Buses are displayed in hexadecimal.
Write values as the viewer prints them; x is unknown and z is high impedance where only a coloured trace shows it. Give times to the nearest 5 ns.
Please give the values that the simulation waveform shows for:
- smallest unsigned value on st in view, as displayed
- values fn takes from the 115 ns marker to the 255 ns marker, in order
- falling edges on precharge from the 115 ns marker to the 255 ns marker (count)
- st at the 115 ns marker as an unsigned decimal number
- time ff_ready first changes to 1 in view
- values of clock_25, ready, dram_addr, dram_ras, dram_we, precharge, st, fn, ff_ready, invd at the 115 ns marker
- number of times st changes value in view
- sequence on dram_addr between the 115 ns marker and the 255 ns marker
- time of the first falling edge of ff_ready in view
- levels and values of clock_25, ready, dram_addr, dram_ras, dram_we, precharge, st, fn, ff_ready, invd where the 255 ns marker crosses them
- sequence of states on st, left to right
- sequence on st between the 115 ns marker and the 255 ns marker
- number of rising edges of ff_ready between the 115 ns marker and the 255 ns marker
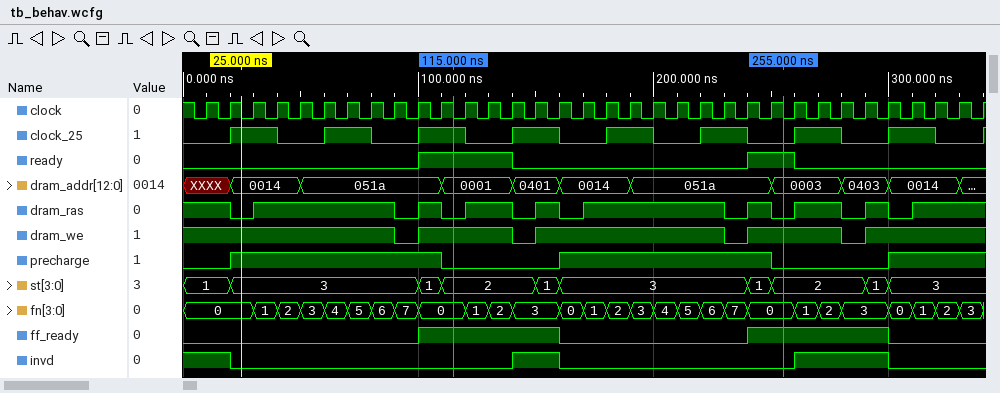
1
0, 1, 2, 3, 0, 1, 2, 3, 4, 5, 6, 7, 0
1
2
100 ns
clock_25=1, ready=1, dram_addr=0001, dram_ras=0, dram_we=1, precharge=0, st=2, fn=0, ff_ready=1, invd=0
9
0001, 0401, 0014, 051a, 0003
160 ns
clock_25=0, ready=1, dram_addr=0003, dram_ras=0, dram_we=1, precharge=0, st=2, fn=0, ff_ready=1, invd=0
1, 3, 1, 2, 1, 3, 1, 2, 1, 3
2, 1, 3, 1, 2
1
